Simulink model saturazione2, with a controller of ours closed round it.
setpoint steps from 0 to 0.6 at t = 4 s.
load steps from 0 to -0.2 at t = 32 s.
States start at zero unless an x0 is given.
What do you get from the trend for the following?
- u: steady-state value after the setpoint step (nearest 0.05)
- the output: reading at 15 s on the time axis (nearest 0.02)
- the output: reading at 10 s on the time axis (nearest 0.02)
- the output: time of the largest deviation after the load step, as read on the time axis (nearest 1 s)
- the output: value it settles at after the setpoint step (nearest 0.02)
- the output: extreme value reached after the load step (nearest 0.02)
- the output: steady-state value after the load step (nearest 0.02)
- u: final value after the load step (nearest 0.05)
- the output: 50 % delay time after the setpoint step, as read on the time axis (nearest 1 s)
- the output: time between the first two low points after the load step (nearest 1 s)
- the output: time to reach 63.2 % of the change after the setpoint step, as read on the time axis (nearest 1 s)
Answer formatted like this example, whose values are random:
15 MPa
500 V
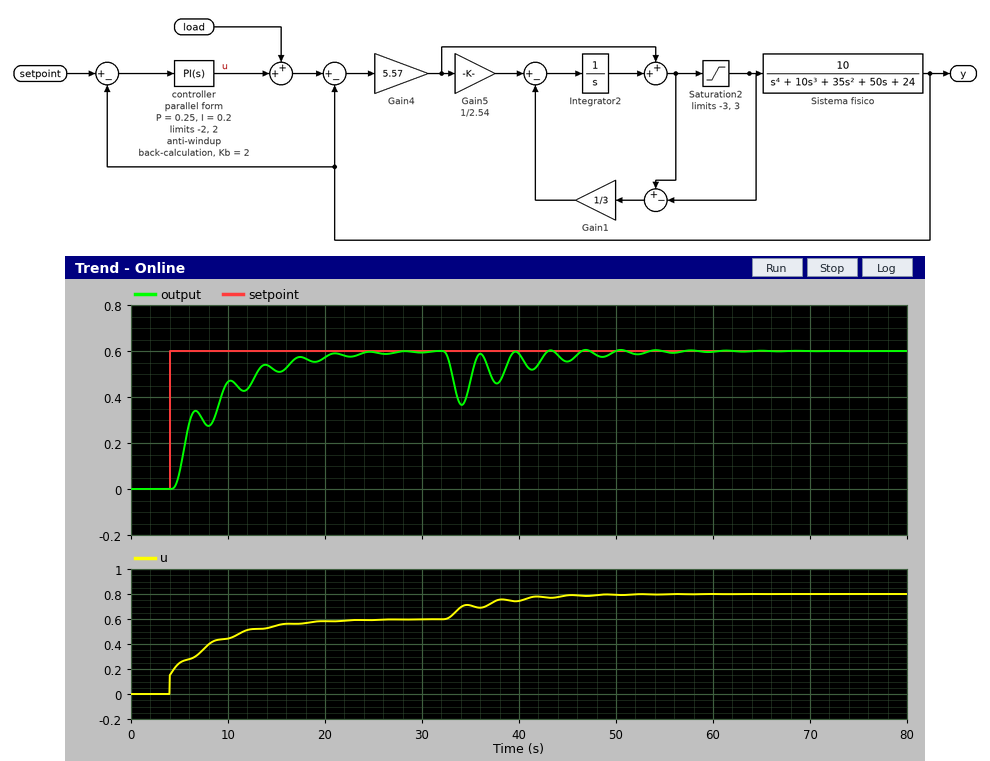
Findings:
0.60
0.52
0.46
34 s
0.60
0.36
0.60
0.80
6 s
4 s
9 s
